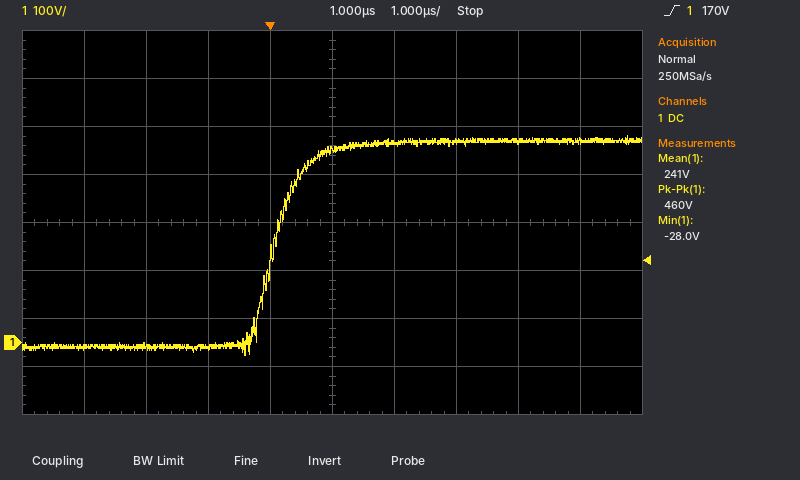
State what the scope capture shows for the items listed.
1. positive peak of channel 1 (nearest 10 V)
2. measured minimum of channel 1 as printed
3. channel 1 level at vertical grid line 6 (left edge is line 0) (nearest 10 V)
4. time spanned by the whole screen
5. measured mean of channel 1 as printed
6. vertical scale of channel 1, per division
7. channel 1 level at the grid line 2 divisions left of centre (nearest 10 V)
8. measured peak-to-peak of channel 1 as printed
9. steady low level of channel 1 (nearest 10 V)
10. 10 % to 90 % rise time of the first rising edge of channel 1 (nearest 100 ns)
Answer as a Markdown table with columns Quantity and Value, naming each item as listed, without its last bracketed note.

| Quantity | Value |
|---|---|
| positive peak of channel 1 | 430 V |
| measured minimum of channel 1 as printed | -28.0 V |
| channel 1 level at vertical grid line 6 (left edge is line 0) | 420 V |
| time spanned by the whole screen | 10 µs |
| measured mean of channel 1 as printed | 241 V |
| vertical scale of channel 1, per division | 100 V |
| channel 1 level at the grid line 2 divisions left of centre | -10 V |
| measured peak-to-peak of channel 1 as printed | 460 V |
| steady low level of channel 1 | -10 V |
| 10 % to 90 % rise time of the first rising edge of channel 1 | 900 ns |
